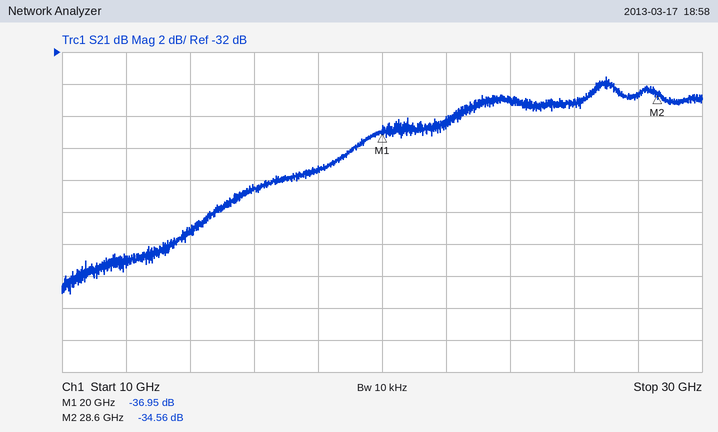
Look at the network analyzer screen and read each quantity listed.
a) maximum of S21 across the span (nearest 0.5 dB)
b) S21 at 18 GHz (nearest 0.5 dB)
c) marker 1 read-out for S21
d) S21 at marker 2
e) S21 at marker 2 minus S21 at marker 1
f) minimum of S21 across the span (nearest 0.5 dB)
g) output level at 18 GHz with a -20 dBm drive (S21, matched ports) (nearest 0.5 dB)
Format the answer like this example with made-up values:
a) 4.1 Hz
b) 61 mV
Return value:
a) -33.5 dB
b) -39.5 dB
c) -36.95 dB
d) -34.56 dB
e) 2.39 dB
f) -47.0 dB
g) -59.5 dBm
